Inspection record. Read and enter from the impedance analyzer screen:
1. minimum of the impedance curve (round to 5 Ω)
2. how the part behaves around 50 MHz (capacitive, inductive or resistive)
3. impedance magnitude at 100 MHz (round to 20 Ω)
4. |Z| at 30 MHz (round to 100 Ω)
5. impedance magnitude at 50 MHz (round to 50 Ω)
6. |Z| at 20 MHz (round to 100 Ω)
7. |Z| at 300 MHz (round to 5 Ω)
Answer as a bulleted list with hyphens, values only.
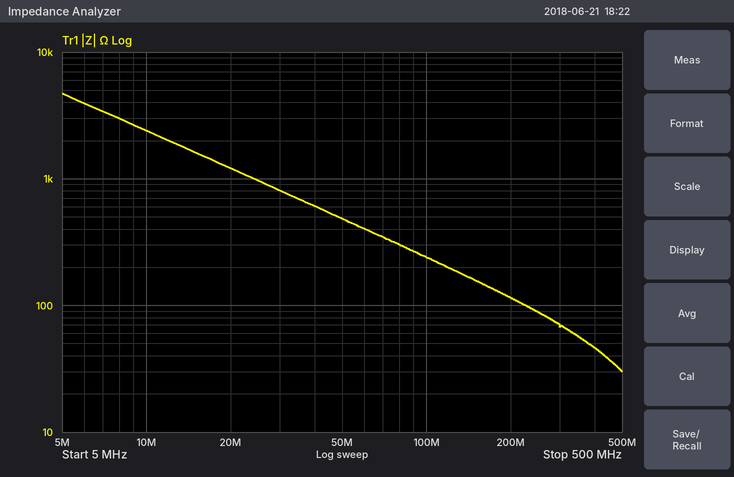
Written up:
- 30 Ω
- capacitive
- 240 Ω
- 800 Ω
- 500 Ω
- 1.2 kΩ
- 70 Ω
